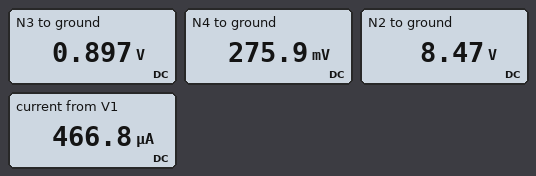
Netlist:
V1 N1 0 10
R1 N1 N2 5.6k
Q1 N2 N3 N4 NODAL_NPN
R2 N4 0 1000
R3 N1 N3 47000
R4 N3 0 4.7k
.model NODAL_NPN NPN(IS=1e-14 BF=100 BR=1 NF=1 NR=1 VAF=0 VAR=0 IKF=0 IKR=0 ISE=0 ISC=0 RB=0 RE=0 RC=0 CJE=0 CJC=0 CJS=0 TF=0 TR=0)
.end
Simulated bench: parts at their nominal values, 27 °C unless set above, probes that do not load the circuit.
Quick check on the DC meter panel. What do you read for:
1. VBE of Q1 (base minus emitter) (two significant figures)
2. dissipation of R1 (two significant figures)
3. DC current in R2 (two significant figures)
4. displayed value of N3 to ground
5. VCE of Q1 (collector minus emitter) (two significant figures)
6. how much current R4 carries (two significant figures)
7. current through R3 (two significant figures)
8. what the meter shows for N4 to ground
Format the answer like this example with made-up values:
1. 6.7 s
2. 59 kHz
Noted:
1. 620 mV
2. 420 µW
3. 280 µA
4. 0.897 V
5. 8.2 V
6. 190 µA
7. 190 µA
8. 275.9 mV
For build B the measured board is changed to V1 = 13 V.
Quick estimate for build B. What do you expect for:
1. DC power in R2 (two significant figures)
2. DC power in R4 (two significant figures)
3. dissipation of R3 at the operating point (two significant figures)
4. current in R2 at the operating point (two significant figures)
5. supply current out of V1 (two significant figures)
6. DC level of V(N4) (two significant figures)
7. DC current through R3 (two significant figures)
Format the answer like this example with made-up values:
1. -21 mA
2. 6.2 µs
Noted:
1. 270 µW
2. 290 µW
3. 3.0 mW
4. 520 µA
5. 770 µA
6. 520 mV
7. 250 µA
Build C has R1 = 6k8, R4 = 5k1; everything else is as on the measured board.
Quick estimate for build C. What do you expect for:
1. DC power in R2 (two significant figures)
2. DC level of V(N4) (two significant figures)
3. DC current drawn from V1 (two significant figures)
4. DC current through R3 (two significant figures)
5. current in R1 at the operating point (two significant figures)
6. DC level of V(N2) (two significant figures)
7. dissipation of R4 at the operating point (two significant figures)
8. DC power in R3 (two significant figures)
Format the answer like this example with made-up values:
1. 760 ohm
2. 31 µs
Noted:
1. 110 µW
2. 340 mV
3. 530 µA
4. 190 µA
5. 330 µA
6. 7.7 V
7. 180 µW
8. 1.7 mW
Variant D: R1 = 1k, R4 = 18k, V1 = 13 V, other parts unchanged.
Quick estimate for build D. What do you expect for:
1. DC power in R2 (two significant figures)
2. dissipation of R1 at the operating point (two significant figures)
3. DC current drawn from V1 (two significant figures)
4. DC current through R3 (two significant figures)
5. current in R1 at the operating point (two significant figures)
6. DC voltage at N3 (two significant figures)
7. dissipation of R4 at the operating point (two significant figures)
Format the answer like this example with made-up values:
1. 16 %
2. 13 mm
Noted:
1. 6.7 mW
2. 6.6 mW
3. 2.8 mA
4. 210 µA
5. 2.6 mA
6. 3.3 V
7. 590 µW
